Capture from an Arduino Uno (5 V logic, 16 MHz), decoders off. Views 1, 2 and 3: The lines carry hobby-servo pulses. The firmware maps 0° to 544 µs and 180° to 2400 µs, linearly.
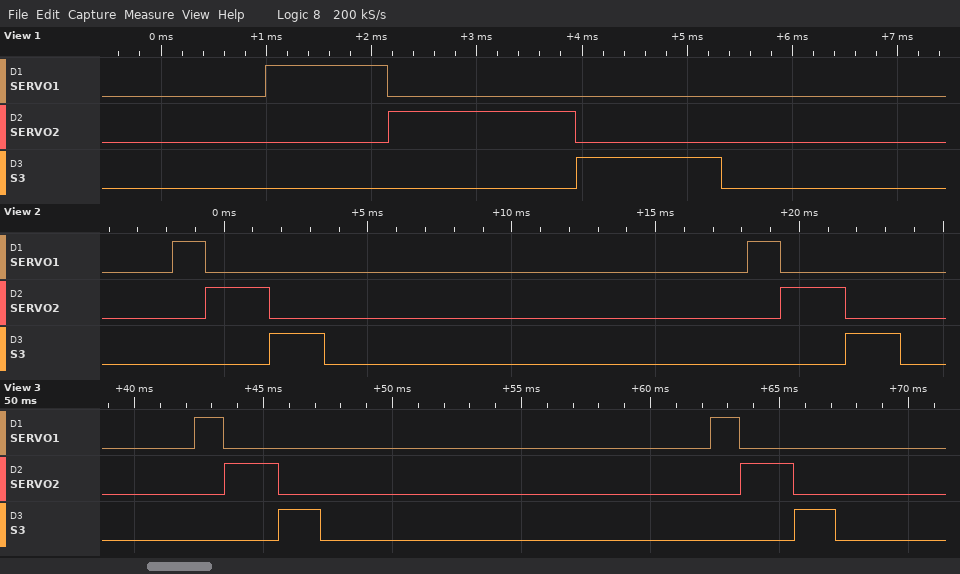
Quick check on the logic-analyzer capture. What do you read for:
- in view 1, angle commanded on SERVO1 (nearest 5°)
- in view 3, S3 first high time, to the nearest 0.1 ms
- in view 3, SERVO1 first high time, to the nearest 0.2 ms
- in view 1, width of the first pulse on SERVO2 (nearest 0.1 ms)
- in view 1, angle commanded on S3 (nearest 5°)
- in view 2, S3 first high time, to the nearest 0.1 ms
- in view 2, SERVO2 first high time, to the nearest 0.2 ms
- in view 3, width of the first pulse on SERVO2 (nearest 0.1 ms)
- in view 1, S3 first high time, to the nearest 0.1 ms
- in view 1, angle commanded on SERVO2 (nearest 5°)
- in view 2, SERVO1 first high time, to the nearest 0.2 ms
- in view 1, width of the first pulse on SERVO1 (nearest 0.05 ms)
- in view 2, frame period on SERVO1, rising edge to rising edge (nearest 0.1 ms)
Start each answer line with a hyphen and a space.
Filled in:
- 60°
- 1.6 ms
- 1.2 ms
- 1.8 ms
- 80°
- 1.9 ms
- 2.2 ms
- 2.1 ms
- 1.4 ms
- 120°
- 1.2 ms
- 1.15 ms
- 20.0 ms
